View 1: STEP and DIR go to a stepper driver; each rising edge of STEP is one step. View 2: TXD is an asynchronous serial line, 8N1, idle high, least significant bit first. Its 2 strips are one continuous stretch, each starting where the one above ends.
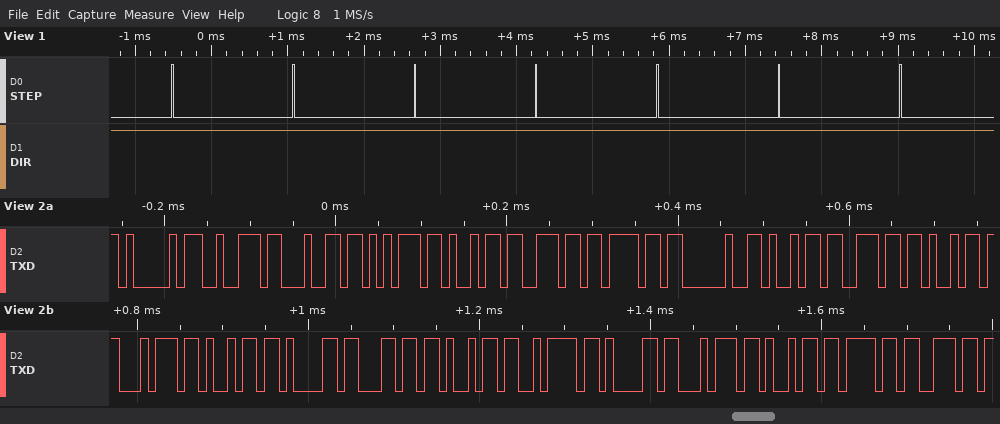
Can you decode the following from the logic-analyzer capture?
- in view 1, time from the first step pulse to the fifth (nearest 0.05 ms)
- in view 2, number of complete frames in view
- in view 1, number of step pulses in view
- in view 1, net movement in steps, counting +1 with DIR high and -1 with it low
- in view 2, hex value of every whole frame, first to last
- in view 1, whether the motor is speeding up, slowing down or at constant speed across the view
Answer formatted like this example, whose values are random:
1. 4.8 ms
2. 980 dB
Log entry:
1. 6.35 ms
2. 22
3. 7
4. +7
5. 41 72 64 75 69 6E 6F 20 69 6E 69 74 69 61 6C 69 7A 61 74 69 6F 6E
6. constant speed
